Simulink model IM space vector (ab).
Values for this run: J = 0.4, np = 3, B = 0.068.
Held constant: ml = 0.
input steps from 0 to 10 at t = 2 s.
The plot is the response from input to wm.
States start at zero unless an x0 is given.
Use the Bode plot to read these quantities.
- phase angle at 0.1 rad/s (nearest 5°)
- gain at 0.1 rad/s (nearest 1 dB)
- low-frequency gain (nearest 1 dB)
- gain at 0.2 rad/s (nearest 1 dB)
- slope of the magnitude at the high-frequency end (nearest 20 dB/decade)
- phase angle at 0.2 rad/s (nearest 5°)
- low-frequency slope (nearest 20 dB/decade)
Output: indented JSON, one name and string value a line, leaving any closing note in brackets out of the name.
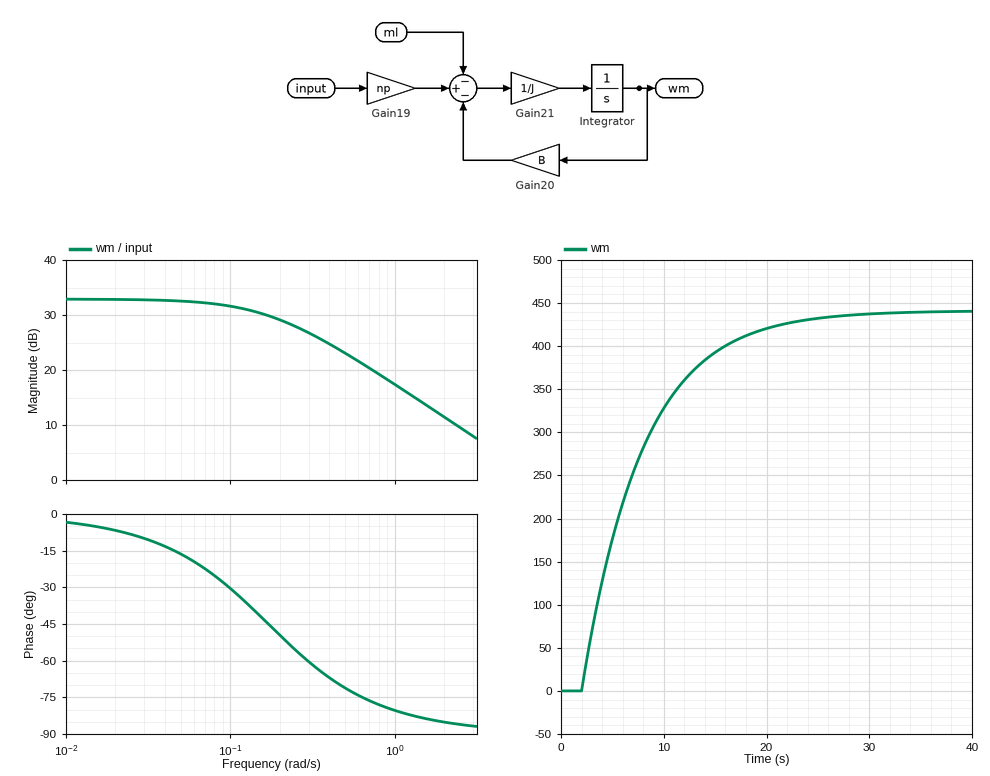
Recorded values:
{
  "phase angle at 0.1 rad/s": "-30°",
  "gain at 0.1 rad/s": "32 dB",
  "low-frequency gain": "33 dB",
  "gain at 0.2 rad/s": "29 dB",
  "slope of the magnitude at the high-frequency end": "-20 dB/decade",
  "phase angle at 0.2 rad/s": "-50°",
  "low-frequency slope": "0 dB/decade"
}
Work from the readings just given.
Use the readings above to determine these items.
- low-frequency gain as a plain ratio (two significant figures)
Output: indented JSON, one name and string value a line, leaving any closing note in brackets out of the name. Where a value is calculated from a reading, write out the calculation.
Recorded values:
{
  "low-frequency gain as a plain ratio": "10^(33 / 20) = 45"
}
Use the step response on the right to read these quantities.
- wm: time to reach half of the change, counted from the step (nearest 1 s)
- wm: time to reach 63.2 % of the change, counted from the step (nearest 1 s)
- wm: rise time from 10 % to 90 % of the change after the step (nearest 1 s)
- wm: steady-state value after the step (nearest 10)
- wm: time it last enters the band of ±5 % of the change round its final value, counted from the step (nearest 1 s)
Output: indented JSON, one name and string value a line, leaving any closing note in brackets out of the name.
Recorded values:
{
  "wm: time to reach half of the change, counted from the step": "4 s",
  "wm: time to reach 63.2 % of the change, counted from the step": "6 s",
  "wm: rise time from 10 % to 90 % of the change after the step": "13 s",
  "wm: steady-state value after the step": "440",
  "wm: time it last enters the band of ±5 % of the change round its final value, counted from the step": "18 s"
}
